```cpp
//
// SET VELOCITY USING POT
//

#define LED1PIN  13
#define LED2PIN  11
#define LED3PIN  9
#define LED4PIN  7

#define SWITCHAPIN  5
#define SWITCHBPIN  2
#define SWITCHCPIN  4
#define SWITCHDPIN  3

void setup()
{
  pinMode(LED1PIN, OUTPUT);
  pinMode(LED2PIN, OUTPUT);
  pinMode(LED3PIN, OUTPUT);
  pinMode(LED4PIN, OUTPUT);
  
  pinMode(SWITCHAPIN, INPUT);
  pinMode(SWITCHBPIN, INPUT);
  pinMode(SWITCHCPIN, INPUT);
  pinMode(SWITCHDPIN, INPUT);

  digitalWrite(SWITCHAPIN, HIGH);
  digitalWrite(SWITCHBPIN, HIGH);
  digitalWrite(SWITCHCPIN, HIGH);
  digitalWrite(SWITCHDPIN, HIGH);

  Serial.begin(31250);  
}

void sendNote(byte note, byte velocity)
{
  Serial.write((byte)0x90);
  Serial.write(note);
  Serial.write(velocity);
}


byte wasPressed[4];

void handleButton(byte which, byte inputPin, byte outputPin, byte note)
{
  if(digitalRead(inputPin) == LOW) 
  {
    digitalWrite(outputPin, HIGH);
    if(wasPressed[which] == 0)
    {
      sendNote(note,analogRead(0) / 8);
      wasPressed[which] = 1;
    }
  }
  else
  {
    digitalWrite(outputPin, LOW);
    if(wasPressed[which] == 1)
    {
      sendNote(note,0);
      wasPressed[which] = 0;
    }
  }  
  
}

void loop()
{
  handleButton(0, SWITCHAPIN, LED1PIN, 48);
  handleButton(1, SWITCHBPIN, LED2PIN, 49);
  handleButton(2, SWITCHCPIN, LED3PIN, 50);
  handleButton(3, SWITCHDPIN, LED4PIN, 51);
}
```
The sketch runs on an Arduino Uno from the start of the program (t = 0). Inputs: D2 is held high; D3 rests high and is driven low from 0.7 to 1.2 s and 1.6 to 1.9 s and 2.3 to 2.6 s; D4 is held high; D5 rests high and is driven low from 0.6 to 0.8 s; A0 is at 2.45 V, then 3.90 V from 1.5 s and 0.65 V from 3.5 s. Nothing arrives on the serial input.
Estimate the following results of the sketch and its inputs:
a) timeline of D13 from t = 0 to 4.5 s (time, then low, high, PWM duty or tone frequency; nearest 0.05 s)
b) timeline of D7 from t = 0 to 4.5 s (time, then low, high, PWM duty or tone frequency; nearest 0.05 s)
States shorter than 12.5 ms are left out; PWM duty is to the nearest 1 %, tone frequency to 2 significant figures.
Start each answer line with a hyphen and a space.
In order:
- 0 s low; 0.6 s high; 0.8 s low
- 0 s low; 0.7 s high; 1.2 s low; 1.6 s high; 1.9 s low; 2.3 s high; 2.6 s low
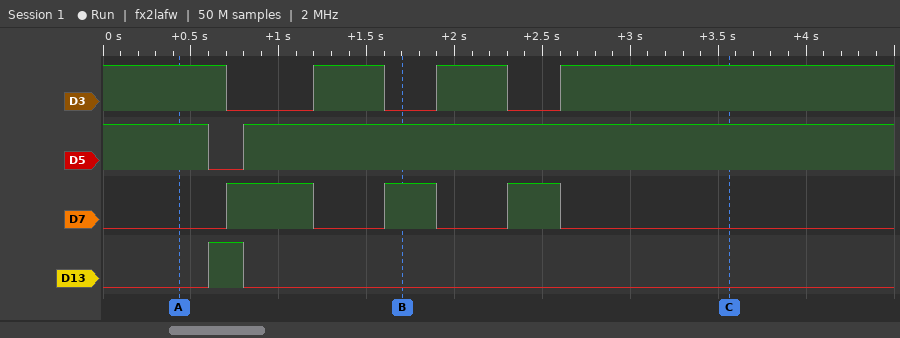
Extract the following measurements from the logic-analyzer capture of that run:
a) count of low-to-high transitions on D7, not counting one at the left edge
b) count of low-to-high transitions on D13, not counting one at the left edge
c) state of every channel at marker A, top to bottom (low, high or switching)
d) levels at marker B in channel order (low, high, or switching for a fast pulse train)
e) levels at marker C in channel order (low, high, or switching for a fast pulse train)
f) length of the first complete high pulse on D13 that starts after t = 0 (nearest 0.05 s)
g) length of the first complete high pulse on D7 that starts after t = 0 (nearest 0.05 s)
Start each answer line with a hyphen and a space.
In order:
- 3
- 1
- D3 high, D5 high, D7 low, D13 low
- D3 low, D5 high, D7 high, D13 low
- D3 high, D5 high, D7 low, D13 low
- 0.20 s
- 0.50 s
